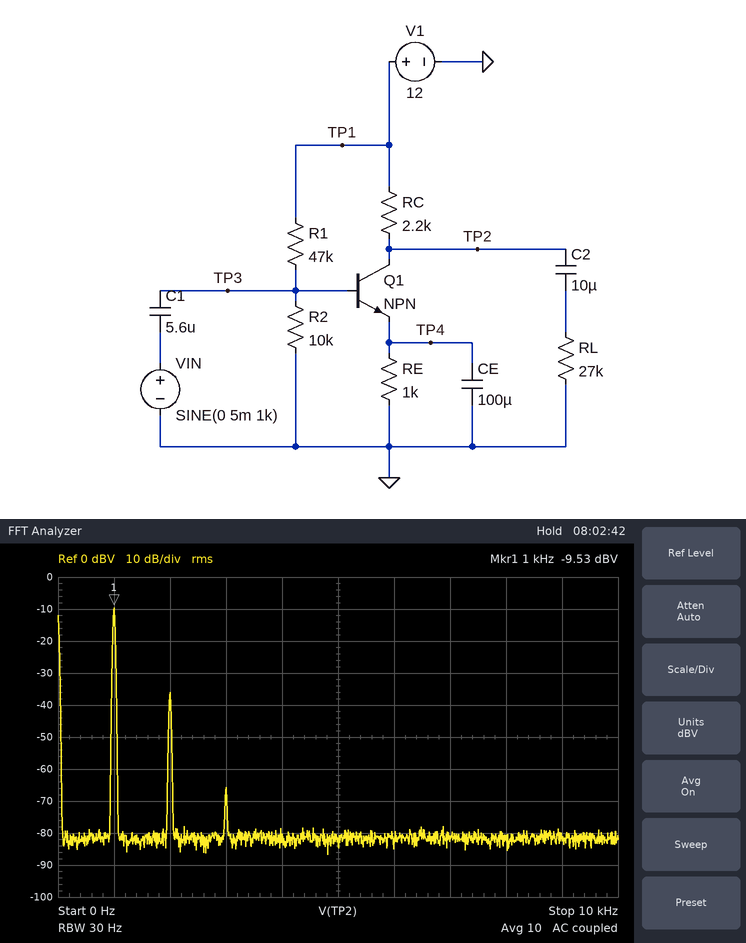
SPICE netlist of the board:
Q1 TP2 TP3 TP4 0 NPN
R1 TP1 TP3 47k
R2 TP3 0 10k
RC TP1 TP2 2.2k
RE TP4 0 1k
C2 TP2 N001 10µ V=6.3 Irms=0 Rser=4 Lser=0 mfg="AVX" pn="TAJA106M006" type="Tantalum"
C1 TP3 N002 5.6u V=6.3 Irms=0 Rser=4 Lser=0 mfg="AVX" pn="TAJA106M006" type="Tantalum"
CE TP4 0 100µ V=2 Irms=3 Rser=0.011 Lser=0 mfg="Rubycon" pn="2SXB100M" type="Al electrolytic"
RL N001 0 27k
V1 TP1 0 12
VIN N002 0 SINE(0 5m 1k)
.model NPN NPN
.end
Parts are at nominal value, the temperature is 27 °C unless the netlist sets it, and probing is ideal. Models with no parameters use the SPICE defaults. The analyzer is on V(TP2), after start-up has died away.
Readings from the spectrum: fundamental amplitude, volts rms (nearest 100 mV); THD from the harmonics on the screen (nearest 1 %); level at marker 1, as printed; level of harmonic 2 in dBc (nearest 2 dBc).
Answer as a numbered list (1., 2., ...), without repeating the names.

1. 300 mV
2. 5 %
3. -9.53 dBV
4. -26 dBc
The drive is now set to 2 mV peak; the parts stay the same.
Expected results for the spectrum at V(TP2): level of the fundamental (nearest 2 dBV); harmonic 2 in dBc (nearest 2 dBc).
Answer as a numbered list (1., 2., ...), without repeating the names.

1. -18 dBV
2. -34 dBc
